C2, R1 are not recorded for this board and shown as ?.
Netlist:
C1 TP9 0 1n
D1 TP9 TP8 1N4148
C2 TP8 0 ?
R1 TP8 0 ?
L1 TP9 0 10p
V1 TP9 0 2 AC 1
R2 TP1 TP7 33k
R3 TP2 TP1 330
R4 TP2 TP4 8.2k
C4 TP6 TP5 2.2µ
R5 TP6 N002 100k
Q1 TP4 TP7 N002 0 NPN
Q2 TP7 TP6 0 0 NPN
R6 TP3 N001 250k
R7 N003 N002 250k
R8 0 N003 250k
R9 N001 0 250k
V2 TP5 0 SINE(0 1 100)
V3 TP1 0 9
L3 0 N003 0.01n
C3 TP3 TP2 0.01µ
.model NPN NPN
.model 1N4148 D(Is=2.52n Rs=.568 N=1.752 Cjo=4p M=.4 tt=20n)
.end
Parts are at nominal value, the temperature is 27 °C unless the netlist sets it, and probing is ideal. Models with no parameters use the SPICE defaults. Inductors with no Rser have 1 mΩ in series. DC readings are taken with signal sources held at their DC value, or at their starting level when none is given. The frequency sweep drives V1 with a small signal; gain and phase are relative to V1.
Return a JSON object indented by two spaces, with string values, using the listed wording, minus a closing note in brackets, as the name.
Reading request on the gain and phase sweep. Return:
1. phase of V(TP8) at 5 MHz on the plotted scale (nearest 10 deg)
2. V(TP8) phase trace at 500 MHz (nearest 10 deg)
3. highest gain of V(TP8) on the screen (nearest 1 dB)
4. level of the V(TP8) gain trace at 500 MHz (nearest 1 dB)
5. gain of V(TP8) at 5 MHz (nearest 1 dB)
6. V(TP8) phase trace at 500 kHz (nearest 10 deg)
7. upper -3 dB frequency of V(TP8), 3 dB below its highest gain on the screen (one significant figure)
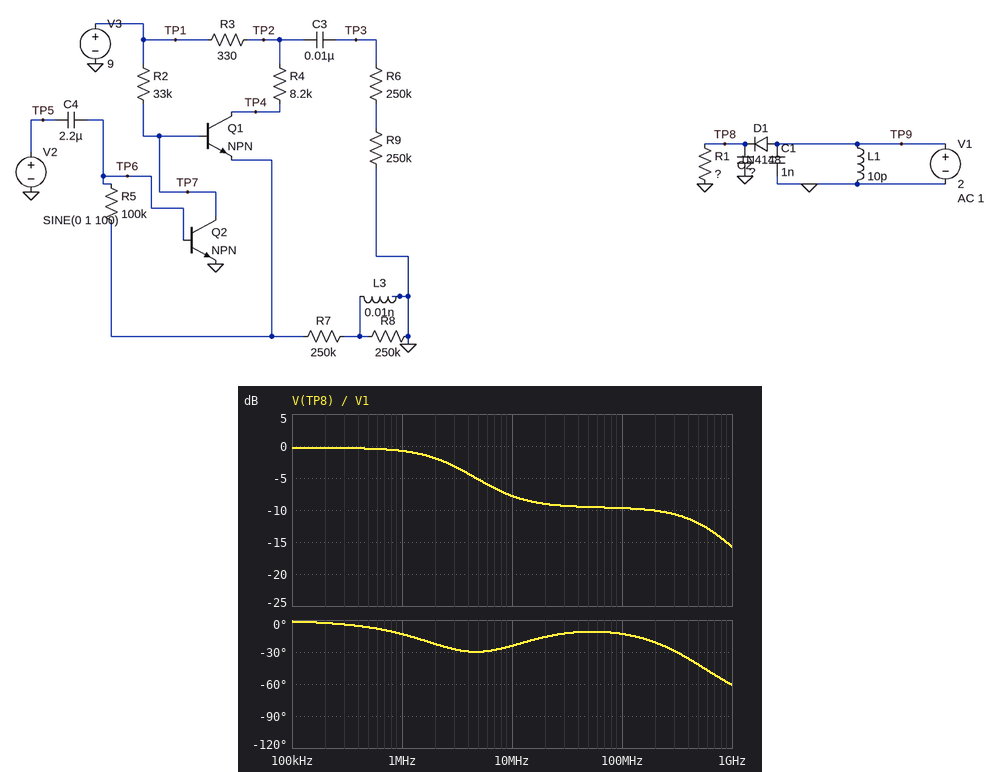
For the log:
{
  "phase of V(TP8) at 5 MHz on the plotted scale": "-30 deg",
  "V(TP8) phase trace at 500 MHz": "-40 deg",
  "highest gain of V(TP8) on the screen": "0 dB",
  "level of the V(TP8) gain trace at 500 MHz": "-12 dB",
  "gain of V(TP8) at 5 MHz": "-5 dB",
  "V(TP8) phase trace at 500 kHz": "-10 deg",
  "upper -3 dB frequency of V(TP8), 3 dB below its highest gain on the screen": "3 MHz"
}
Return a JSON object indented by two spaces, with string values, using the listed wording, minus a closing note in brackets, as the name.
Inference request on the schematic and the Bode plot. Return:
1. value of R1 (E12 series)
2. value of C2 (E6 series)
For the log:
{
  "value of R1": "820 Ω",
  "value of C2": "1.5 nF"
}
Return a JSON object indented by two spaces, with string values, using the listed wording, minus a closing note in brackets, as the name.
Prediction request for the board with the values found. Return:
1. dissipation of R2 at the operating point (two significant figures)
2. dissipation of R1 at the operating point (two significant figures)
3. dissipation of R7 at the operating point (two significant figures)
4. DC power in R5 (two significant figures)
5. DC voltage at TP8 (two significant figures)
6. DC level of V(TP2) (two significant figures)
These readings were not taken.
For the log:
{
  "dissipation of R2 at the operating point": "1.7 mW",
  "dissipation of R1 at the operating point": "2.4 mW",
  "dissipation of R7 at the operating point": "3.7 µW",
  "DC power in R5": "500 nW",
  "DC voltage at TP8": "1.4 V",
  "DC level of V(TP2)": "9.0 V"
}
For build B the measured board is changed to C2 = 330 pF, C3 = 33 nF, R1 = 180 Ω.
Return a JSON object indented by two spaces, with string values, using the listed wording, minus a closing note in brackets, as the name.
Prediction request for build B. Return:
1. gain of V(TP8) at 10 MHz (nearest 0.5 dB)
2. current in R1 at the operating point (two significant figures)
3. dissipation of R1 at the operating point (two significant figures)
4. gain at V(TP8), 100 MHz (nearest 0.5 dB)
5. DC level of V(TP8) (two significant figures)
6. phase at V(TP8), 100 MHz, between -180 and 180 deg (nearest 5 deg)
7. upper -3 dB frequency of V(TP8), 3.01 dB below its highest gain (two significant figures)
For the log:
{
  "gain of V(TP8) at 10 MHz": "-0.5 dB",
  "current in R1 at the operating point": "7.3 mA",
  "dissipation of R1 at the operating point": "9.7 mW",
  "gain at V(TP8), 100 MHz": "-1.0 dB",
  "DC level of V(TP8)": "1.3 V",
  "phase at V(TP8), 100 MHz, between -180 and 180 deg": "-5 deg",
  "upper -3 dB frequency of V(TP8), 3.01 dB below its highest gain": "820 MHz"
}
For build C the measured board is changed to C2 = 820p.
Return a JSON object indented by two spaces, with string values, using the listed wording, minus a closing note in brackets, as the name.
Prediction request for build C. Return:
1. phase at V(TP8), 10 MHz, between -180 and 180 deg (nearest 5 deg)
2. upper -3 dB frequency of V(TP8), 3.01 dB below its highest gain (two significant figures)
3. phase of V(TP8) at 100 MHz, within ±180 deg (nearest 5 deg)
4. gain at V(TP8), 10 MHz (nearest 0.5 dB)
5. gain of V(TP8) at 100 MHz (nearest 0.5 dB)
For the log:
{
  "phase at V(TP8), 10 MHz, between -180 and 180 deg": "-20 deg",
  "upper -3 dB frequency of V(TP8), 3.01 dB below its highest gain": "5.4 MHz",
  "phase of V(TP8) at 100 MHz, within ±180 deg": "-10 deg",
  "gain at V(TP8), 10 MHz": "-5.0 dB",
  "gain of V(TP8) at 100 MHz": "-6.5 dB"
}
